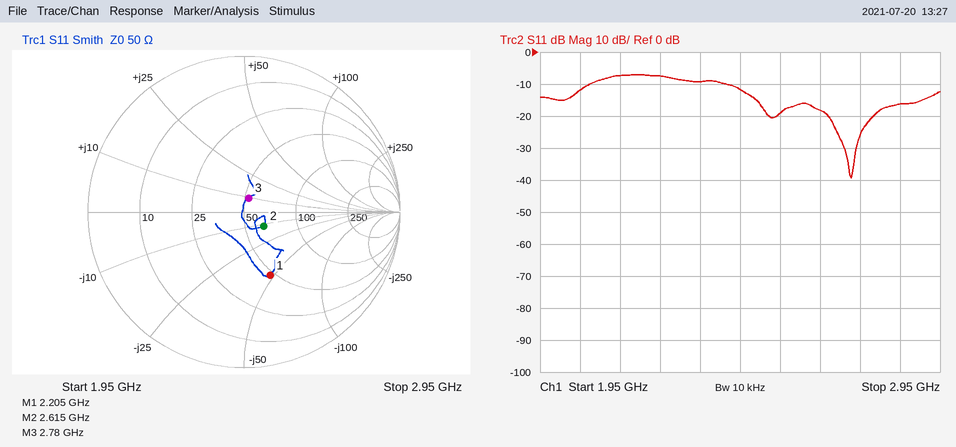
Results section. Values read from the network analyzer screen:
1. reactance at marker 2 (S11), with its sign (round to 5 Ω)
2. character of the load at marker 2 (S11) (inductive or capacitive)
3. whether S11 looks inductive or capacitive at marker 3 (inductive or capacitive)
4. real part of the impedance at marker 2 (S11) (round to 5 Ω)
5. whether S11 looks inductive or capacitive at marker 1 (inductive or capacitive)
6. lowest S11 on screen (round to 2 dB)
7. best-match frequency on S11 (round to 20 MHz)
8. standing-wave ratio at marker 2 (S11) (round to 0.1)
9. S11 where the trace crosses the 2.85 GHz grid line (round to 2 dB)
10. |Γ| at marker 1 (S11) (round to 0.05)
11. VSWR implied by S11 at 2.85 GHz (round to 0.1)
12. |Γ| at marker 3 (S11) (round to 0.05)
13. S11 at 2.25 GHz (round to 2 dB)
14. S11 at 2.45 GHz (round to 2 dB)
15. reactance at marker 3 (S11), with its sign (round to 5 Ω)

-10 Ω
capacitive
inductive
65 Ω
capacitive
-40 dB
2.72 GHz
1.4
-16 dB
0.45
1.4
0.10
-8 dB
-12 dB
+10 Ω
